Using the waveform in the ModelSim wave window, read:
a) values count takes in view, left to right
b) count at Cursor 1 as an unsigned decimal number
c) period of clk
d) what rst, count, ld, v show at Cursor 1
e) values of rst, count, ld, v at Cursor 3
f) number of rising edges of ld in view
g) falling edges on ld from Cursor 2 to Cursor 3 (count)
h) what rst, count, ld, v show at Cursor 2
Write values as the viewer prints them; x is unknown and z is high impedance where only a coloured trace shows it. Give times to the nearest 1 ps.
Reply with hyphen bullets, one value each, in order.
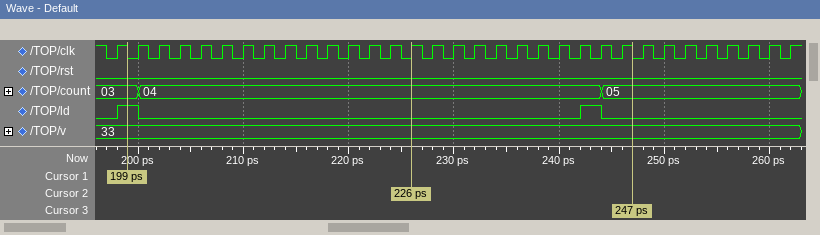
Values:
- 03, 04, 05
- 3
- 2 ps
- rst=0, count=03, ld=1, v=33
- rst=0, count=05, ld=0, v=33
- 2
- 1
- rst=0, count=04, ld=0, v=33
